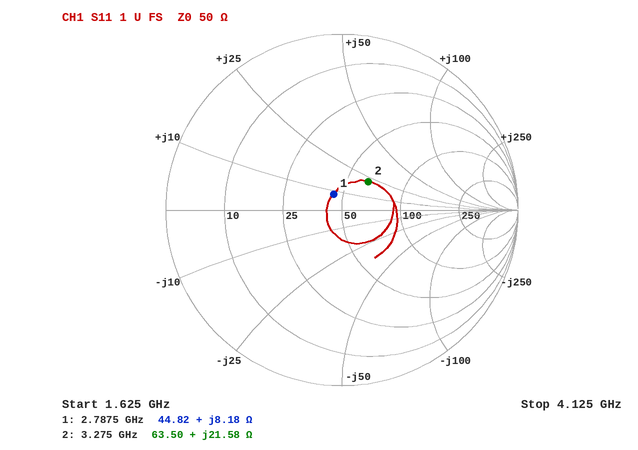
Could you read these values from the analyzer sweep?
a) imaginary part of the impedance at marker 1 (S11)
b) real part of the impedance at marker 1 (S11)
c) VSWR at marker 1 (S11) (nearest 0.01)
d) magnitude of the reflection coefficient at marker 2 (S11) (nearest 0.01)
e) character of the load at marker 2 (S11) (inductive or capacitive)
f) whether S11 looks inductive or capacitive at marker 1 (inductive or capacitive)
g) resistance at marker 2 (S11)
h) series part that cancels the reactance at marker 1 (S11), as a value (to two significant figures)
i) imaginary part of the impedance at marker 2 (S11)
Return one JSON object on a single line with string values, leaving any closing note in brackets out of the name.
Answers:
{"imaginary part of the impedance at marker 1": "+8.18 Ω", "real part of the impedance at marker 1": "44.82 Ω", "VSWR at marker 1 (S11)": "1.23", "magnitude of the reflection coefficient at marker 2 (S11)": "0.22", "character of the load at marker 2 (S11)": "inductive", "whether S11 looks inductive or capacitive at marker 1": "inductive", "resistance at marker 2": "63.50 Ω", "series part that cancels the reactance at marker 1 (S11), as a value": "7.0 pF", "imaginary part of the impedance at marker 2": "+21.58 Ω"}
